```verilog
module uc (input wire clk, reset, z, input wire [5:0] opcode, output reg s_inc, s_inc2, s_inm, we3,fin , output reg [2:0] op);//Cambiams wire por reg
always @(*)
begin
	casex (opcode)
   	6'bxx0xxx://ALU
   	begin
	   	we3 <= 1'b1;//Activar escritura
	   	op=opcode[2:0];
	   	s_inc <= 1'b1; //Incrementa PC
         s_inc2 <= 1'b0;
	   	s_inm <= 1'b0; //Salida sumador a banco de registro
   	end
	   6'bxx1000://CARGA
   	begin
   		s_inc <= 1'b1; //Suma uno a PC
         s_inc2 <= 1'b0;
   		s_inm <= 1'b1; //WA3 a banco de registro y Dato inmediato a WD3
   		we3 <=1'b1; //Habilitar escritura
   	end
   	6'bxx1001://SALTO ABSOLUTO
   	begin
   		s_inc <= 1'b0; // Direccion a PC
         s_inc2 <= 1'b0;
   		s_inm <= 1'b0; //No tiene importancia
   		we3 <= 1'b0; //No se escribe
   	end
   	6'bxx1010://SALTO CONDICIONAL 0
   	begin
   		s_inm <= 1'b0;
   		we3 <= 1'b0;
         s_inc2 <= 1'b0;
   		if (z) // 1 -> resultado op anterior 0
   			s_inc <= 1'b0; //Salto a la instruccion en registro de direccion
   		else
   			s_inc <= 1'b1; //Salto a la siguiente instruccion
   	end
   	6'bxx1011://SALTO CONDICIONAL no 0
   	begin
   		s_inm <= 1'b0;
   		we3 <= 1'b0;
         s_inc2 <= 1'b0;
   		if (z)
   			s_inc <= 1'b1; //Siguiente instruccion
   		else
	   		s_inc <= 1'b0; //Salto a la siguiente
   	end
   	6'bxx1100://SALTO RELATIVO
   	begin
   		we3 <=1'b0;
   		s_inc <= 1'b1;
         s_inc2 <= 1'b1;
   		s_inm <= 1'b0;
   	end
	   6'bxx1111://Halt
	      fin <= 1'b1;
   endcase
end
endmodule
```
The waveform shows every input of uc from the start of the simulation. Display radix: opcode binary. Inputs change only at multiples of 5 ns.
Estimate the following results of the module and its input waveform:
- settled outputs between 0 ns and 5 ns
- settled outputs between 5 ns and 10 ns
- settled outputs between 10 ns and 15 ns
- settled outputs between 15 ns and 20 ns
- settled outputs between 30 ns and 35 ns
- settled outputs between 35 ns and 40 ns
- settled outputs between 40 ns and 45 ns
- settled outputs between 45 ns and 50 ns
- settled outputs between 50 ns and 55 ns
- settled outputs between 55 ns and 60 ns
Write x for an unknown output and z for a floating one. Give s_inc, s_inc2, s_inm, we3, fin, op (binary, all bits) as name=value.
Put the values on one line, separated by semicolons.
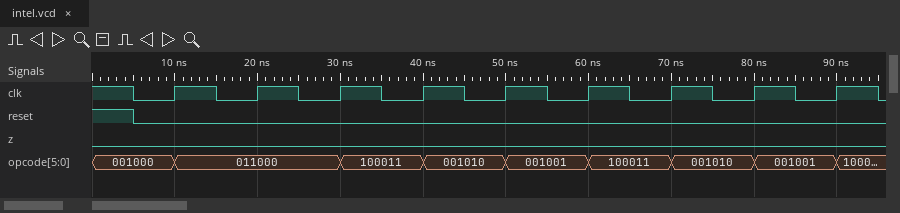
s_inc=1, s_inc2=0, s_inm=1, we3=1, fin=x, op=x; s_inc=1, s_inc2=0, s_inm=1, we3=1, fin=x, op=x; s_inc=1, s_inc2=0, s_inm=1, we3=1, fin=x, op=x; s_inc=1, s_inc2=0, s_inm=1, we3=1, fin=x, op=x; s_inc=1, s_inc2=0, s_inm=0, we3=1, fin=x, op=011; s_inc=1, s_inc2=0, s_inm=0, we3=1, fin=x, op=011; s_inc=1, s_inc2=0, s_inm=0, we3=0, fin=x, op=011; s_inc=1, s_inc2=0, s_inm=0, we3=0, fin=x, op=011; s_inc=0, s_inc2=0, s_inm=0, we3=0, fin=x, op=011; s_inc=0, s_inc2=0, s_inm=0, we3=0, fin=x, op=011
